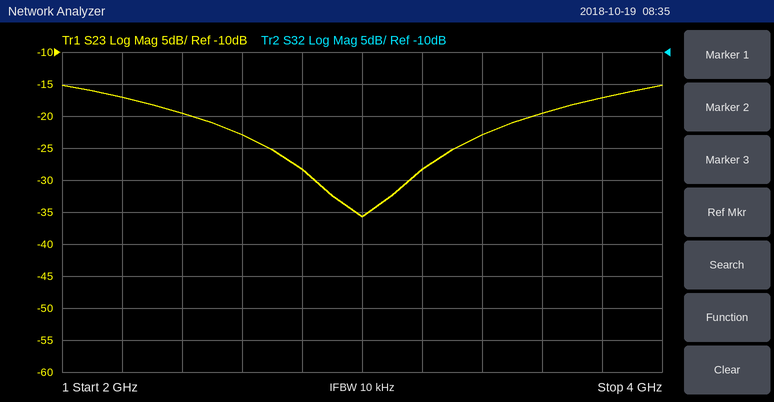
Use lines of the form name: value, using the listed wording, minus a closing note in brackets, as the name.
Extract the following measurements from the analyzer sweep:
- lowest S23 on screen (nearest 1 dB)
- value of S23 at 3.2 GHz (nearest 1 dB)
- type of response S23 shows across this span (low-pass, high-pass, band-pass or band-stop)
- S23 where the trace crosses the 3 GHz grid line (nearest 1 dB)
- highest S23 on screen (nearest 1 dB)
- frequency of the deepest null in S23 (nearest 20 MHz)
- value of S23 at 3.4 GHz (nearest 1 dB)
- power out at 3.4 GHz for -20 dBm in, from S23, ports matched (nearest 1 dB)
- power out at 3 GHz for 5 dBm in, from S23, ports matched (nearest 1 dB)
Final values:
lowest S23 on screen: -36 dB
value of S23 at 3.2 GHz: -28 dB
type of response S23 shows across this span: band-stop
S23 where the trace crosses the 3 GHz grid line: -36 dB
highest S23 on screen: -15 dB
frequency of the deepest null in S23: 3.00 GHz
value of S23 at 3.4 GHz: -23 dB
power out at 3.4 GHz for -20 dBm in, from S23, ports matched: -43 dBm
power out at 3 GHz for 5 dBm in, from S23, ports matched: -31 dBm
